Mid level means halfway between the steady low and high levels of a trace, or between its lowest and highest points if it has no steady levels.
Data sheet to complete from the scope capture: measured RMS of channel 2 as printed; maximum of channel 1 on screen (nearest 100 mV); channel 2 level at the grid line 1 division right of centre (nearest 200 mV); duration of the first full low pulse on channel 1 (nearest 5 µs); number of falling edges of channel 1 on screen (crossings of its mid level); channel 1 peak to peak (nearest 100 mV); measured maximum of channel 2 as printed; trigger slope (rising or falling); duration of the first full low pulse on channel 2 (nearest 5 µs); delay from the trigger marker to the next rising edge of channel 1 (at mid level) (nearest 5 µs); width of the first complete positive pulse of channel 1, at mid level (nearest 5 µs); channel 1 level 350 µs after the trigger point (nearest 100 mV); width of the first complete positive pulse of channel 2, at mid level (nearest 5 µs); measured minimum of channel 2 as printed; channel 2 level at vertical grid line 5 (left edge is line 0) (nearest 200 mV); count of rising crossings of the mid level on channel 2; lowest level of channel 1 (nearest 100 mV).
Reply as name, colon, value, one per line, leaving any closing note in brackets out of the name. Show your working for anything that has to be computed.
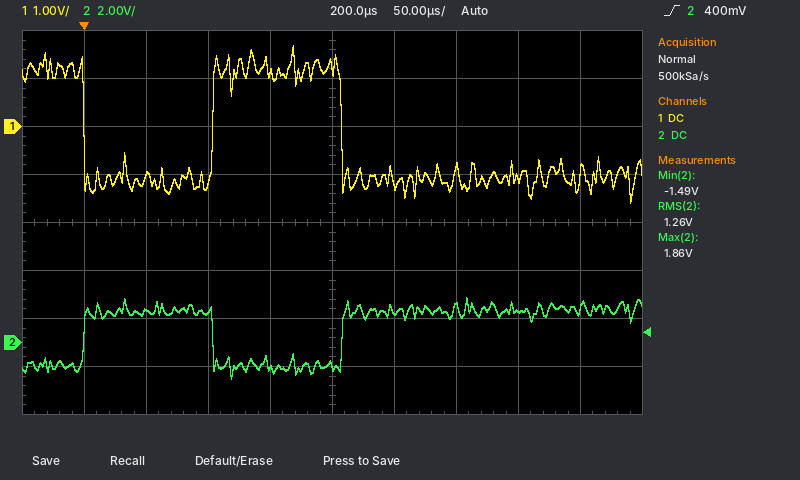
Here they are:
measured RMS of channel 2 as printed: 1.26 V
maximum of channel 1 on screen: 1.7 V
channel 2 level at the grid line 1 division right of centre: 1.4 V
duration of the first full low pulse on channel 1: 105 µs
number of falling edges of channel 1 on screen: 2
channel 1 peak to peak: 1.7 V − (-1.6 V) = 3.3 V
measured maximum of channel 2 as printed: 1.86 V
trigger slope: rising
duration of the first full low pulse on channel 2: 105 µs
delay from the trigger marker to the next rising edge of channel 1 (at mid level): 105 µs
width of the first complete positive pulse of channel 1, at mid level: 105 µs
channel 1 level 350 µs after the trigger point: -1.1 V
width of the first complete positive pulse of channel 2, at mid level: 105 µs
measured minimum of channel 2 as printed: -1.49 V
channel 2 level at vertical grid line 5 (left edge is line 0): -1.0 V
count of rising crossings of the mid level on channel 2: 2
lowest level of channel 1: -1.6 V
